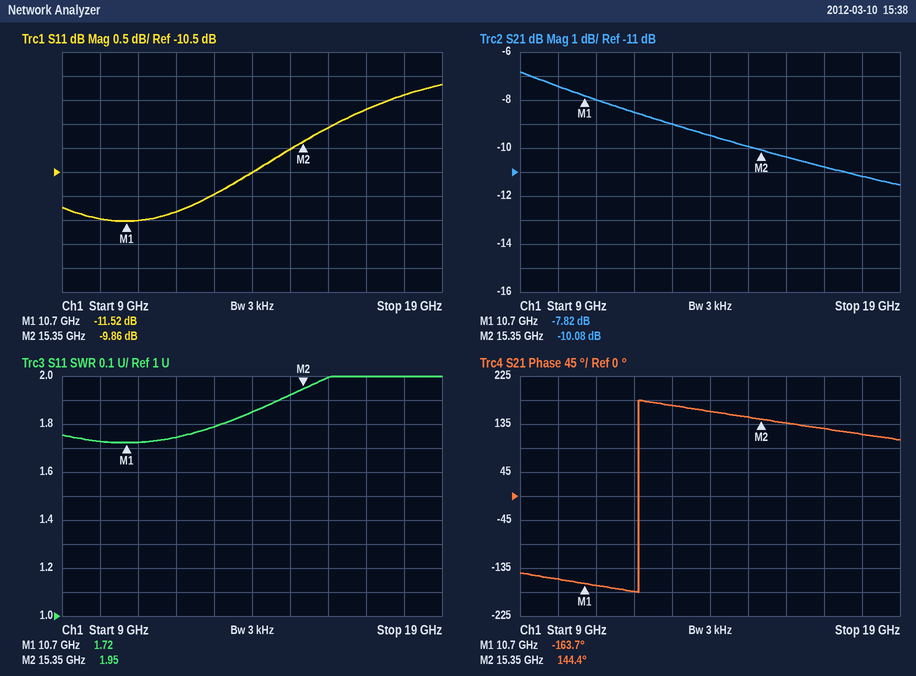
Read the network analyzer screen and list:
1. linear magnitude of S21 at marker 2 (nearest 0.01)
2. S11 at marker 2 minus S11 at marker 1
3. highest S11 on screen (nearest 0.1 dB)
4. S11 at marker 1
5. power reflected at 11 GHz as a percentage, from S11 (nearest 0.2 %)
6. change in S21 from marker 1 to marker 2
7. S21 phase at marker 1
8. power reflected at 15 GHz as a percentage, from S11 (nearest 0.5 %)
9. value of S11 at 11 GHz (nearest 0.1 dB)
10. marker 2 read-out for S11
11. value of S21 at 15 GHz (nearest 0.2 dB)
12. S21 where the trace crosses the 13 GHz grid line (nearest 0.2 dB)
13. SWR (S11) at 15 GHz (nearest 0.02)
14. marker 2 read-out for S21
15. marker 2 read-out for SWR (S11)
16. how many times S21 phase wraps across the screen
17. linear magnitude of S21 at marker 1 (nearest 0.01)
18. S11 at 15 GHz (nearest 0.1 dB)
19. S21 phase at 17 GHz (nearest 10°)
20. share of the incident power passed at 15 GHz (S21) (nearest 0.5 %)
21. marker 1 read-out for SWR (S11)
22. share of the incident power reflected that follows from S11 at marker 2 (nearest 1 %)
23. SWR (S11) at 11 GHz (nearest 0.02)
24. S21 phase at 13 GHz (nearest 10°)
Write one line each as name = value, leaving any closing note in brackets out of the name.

linear magnitude of S21 at marker 2 = 0.31
S11 at marker 2 minus S11 at marker 1 = 1.66 dB
highest S11 on screen = -8.7 dB
S11 at marker 1 = -11.52 dB
power reflected at 11 GHz as a percentage, from S11 = 7.0 %
change in S21 from marker 1 to marker 2 = -2.26 dB
S21 phase at marker 1 = -163.7°
power reflected at 15 GHz as a percentage, from S11 = 10.0 %
value of S11 at 11 GHz = -11.5 dB
marker 2 read-out for S11 = -9.86 dB
value of S21 at 15 GHz = -10.0 dB
S21 where the trace crosses the 13 GHz grid line = -9.0 dB
SWR (S11) at 15 GHz = 1.92
marker 2 read-out for S21 = -10.08 dB
marker 2 read-out for SWR = 1.95
how many times S21 phase wraps across the screen = 1
linear magnitude of S21 at marker 1 = 0.41
S11 at 15 GHz = -10.0 dB
S21 phase at 17 GHz = 130°
share of the incident power passed at 15 GHz (S21) = 10.0 %
marker 1 read-out for SWR = 1.72
share of the incident power reflected that follows from S11 at marker 2 = 10 %
SWR (S11) at 11 GHz = 1.72
S21 phase at 13 GHz = 170°
